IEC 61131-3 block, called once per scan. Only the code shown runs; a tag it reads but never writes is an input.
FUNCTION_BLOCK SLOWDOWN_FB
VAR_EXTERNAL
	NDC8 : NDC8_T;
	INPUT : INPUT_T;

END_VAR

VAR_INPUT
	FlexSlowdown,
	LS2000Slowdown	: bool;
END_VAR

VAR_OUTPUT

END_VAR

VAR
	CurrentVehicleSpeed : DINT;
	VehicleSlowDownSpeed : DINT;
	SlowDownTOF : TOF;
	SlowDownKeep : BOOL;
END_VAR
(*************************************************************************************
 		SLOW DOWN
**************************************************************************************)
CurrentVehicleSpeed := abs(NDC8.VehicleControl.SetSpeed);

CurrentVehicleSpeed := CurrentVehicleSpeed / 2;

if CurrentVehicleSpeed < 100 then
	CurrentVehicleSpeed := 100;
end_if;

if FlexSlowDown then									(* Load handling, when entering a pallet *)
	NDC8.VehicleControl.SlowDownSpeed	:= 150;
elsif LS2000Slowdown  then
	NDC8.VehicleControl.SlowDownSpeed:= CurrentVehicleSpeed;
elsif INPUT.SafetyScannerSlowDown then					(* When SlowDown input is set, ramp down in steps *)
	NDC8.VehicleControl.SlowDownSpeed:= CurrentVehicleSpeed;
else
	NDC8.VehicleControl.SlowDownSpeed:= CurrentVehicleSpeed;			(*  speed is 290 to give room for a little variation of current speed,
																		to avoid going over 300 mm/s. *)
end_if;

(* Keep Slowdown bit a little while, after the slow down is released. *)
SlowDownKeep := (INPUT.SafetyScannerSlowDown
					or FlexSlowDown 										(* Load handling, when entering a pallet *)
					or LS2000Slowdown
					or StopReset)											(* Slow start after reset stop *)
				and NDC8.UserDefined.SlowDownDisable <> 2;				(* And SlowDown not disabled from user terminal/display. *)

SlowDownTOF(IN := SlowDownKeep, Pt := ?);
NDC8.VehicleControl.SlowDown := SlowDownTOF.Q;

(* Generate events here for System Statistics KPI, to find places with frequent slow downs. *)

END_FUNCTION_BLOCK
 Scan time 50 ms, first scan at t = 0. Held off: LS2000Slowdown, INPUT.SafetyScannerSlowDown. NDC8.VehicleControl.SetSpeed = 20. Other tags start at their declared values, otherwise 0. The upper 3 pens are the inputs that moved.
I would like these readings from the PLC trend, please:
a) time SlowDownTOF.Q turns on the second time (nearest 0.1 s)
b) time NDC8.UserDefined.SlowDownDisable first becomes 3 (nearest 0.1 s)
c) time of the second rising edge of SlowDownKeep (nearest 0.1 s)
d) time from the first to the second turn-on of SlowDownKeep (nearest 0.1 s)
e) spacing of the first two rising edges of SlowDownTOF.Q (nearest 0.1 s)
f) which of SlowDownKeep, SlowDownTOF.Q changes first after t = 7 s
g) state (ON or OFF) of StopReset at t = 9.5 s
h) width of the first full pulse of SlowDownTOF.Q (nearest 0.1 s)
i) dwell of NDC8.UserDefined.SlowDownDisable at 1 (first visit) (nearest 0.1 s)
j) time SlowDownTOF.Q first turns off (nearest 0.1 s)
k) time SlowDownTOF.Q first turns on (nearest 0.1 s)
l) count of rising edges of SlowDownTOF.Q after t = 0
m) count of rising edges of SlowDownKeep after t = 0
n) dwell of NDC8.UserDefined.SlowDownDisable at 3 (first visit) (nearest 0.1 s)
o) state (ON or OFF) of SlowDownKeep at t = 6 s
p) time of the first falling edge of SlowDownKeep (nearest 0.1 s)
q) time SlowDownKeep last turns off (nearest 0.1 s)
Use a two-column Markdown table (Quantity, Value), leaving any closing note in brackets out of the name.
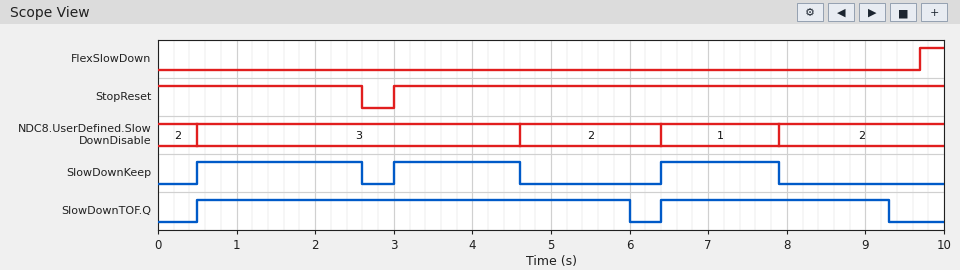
| Quantity | Value |
|---|---|
| time SlowDownTOF.Q turns on the second time | 6.4 s |
| time NDC8.UserDefined.SlowDownDisable first becomes 3 | 0.5 s |
| time of the second rising edge of SlowDownKeep | 3.0 s |
| time from the first to the second turn-on of SlowDownKeep | 2.5 s |
| spacing of the first two rising edges of SlowDownTOF.Q | 5.9 s |
| which of SlowDownKeep, SlowDownTOF.Q changes first after t = 7 s | SlowDownKeep |
| state (ON or OFF) of StopReset at t = 9.5 s | ON |
| width of the first full pulse of SlowDownTOF.Q | 5.5 s |
| dwell of NDC8.UserDefined.SlowDownDisable at 1 (first visit) | 1.5 s |
| time SlowDownTOF.Q first turns off | 6.0 s |
| time SlowDownTOF.Q first turns on | 0.5 s |
| count of rising edges of SlowDownTOF.Q after t = 0 | 2 |
| count of rising edges of SlowDownKeep after t = 0 | 3 |
| dwell of NDC8.UserDefined.SlowDownDisable at 3 (first visit) | 4.1 s |
| state (ON or OFF) of SlowDownKeep at t = 6 s | OFF |
| time of the first falling edge of SlowDownKeep | 2.6 s |
| time SlowDownKeep last turns off | 7.9 s |
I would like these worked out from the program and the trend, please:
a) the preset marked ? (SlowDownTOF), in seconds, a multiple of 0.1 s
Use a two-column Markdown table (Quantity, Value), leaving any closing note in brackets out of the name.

| Quantity | Value |
|---|---|
| the preset marked ? (SlowDownTOF), in seconds, a multiple of 0.1 s | 1.4 s |
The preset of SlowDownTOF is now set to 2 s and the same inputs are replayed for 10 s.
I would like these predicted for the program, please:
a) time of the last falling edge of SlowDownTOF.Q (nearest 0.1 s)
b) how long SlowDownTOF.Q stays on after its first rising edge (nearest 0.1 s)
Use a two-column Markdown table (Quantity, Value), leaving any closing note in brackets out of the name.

| Quantity | Value |
|---|---|
| time of the last falling edge of SlowDownTOF.Q | 9.9 s |
| how long SlowDownTOF.Q stays on after its first rising edge | 9.4 s |
